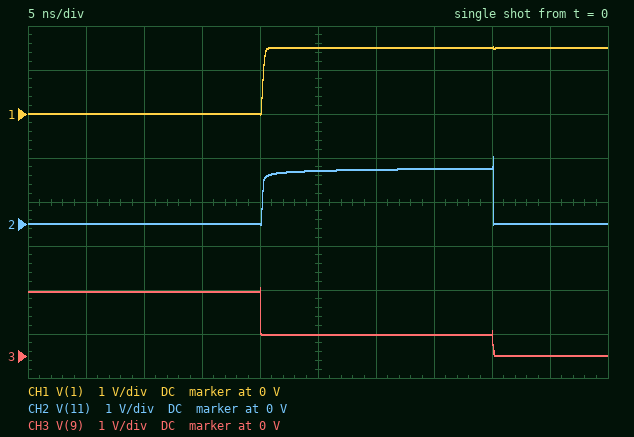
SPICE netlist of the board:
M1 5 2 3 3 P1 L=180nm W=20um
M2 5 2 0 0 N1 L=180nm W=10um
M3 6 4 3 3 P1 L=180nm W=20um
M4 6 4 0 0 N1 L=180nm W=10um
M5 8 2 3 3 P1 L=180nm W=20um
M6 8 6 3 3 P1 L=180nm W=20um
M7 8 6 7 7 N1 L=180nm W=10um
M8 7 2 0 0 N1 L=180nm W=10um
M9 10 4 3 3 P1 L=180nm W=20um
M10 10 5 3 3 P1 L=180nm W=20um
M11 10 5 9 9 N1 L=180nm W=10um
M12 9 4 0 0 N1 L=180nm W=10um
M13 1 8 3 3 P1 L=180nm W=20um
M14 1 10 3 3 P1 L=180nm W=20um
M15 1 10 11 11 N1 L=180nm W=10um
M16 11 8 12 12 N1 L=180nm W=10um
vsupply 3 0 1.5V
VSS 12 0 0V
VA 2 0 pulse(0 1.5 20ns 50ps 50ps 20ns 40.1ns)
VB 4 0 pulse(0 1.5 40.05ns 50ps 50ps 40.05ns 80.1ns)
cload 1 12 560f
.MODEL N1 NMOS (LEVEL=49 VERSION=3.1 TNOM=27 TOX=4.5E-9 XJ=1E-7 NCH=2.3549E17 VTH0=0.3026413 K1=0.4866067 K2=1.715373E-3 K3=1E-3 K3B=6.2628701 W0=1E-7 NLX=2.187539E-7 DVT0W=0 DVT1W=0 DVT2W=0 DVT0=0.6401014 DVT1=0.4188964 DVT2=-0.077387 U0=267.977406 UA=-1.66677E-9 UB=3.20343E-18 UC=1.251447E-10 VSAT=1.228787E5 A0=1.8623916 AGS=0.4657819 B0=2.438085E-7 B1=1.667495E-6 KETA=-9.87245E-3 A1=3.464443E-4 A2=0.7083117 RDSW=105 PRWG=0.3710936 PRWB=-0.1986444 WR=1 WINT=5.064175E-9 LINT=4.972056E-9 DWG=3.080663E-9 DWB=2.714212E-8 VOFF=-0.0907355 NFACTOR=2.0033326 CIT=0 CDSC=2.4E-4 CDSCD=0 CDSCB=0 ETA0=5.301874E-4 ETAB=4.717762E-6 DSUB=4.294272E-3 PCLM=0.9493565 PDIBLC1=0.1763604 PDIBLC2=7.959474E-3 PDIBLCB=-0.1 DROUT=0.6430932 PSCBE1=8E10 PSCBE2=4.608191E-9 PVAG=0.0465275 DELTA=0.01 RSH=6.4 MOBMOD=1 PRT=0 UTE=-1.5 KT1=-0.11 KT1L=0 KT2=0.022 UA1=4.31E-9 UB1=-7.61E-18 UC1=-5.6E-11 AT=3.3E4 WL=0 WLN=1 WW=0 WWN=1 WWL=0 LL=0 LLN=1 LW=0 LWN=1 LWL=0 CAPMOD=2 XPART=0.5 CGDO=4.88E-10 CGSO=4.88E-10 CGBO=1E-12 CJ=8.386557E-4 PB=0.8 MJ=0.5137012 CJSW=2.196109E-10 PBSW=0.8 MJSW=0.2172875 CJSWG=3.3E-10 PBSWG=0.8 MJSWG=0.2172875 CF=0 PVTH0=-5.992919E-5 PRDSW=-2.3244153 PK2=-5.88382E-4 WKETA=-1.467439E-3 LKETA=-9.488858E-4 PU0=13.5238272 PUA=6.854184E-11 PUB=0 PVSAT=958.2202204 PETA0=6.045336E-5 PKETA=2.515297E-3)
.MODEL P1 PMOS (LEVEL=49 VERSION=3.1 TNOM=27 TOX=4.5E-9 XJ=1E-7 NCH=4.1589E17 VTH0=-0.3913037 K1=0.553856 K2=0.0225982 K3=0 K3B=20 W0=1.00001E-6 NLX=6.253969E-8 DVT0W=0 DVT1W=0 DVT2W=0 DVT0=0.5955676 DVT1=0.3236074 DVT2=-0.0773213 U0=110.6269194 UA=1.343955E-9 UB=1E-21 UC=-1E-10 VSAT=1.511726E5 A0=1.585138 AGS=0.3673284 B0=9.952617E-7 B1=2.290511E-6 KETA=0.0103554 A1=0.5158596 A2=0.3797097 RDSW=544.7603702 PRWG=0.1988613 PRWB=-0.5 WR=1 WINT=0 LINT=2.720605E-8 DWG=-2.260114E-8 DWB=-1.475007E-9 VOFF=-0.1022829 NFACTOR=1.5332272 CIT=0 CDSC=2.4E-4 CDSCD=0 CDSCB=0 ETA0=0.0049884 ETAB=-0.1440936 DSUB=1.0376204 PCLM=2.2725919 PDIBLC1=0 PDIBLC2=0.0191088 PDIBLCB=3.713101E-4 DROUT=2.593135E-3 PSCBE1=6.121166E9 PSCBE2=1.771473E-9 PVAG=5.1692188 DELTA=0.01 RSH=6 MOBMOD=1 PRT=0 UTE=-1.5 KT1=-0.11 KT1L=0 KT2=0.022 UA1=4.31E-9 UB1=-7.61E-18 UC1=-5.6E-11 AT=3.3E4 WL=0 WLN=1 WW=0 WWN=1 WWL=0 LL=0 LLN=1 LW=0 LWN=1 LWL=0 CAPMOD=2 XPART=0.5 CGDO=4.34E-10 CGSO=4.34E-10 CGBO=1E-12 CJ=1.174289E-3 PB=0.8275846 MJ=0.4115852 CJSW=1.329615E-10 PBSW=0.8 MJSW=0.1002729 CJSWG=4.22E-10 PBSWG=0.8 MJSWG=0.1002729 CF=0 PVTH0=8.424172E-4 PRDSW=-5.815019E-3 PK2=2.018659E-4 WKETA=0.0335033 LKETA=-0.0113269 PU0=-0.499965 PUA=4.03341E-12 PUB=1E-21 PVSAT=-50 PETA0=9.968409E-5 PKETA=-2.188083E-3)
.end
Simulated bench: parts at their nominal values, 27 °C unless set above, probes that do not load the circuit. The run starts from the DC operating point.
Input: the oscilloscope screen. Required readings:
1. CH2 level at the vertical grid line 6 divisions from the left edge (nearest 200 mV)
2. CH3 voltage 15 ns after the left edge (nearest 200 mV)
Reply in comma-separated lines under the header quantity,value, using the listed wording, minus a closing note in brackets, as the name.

quantity,value
CH2 level at the vertical grid line 6 divisions from the left edge,1.2 V
CH3 voltage 15 ns after the left edge,1.4 V
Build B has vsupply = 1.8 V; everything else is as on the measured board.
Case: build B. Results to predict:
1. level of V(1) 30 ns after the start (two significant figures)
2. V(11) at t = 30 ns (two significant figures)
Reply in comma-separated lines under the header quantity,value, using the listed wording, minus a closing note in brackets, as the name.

quantity,value
level of V(1) 30 ns after the start,1.8 V
V(11) at t = 30 ns,1.5 V
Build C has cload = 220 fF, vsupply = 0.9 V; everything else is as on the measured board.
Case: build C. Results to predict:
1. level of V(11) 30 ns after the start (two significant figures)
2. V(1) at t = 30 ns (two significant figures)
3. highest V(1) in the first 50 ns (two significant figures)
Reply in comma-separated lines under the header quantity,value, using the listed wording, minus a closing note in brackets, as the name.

quantity,value
level of V(11) 30 ns after the start,630 mV
V(1) at t = 30 ns,900 mV
highest V(1) in the first 50 ns,960 mV
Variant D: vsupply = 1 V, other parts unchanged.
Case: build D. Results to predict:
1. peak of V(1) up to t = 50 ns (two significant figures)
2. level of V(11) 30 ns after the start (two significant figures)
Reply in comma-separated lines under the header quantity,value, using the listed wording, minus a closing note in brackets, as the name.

quantity,value
peak of V(1) up to t = 50 ns,1.0 V
level of V(11) 30 ns after the start,730 mV
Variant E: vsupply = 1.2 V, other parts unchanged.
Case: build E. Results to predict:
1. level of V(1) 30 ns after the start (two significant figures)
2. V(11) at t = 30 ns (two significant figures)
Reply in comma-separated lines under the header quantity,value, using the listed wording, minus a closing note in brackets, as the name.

quantity,value
level of V(1) 30 ns after the start,1.2 V
V(11) at t = 30 ns,930 mV
